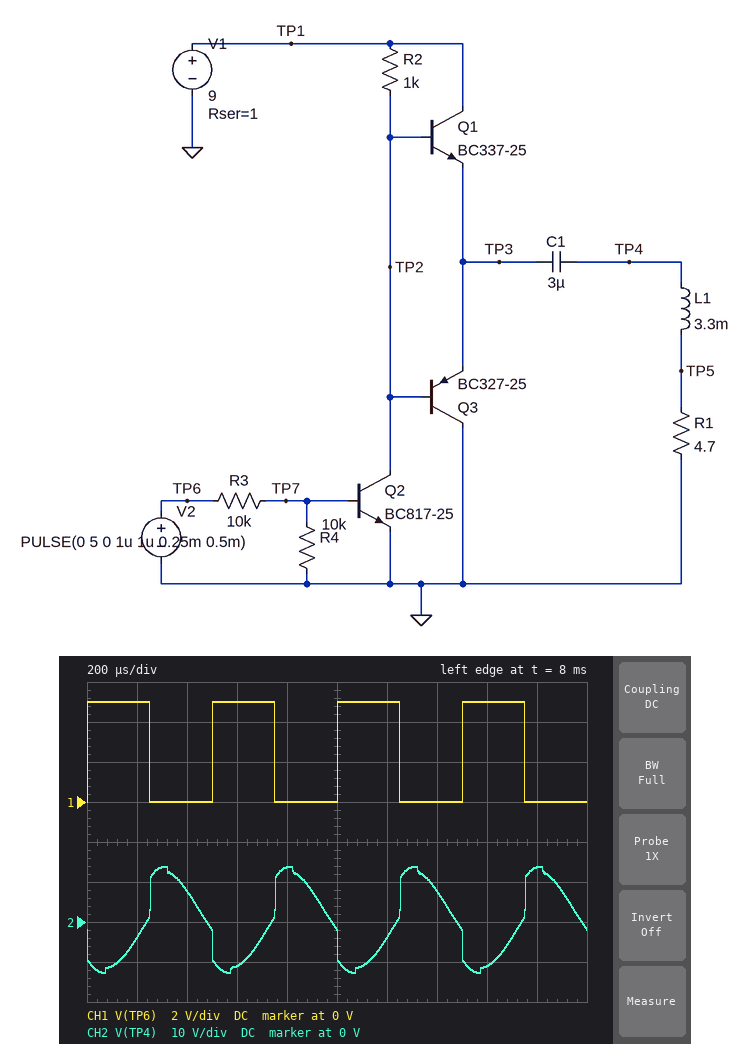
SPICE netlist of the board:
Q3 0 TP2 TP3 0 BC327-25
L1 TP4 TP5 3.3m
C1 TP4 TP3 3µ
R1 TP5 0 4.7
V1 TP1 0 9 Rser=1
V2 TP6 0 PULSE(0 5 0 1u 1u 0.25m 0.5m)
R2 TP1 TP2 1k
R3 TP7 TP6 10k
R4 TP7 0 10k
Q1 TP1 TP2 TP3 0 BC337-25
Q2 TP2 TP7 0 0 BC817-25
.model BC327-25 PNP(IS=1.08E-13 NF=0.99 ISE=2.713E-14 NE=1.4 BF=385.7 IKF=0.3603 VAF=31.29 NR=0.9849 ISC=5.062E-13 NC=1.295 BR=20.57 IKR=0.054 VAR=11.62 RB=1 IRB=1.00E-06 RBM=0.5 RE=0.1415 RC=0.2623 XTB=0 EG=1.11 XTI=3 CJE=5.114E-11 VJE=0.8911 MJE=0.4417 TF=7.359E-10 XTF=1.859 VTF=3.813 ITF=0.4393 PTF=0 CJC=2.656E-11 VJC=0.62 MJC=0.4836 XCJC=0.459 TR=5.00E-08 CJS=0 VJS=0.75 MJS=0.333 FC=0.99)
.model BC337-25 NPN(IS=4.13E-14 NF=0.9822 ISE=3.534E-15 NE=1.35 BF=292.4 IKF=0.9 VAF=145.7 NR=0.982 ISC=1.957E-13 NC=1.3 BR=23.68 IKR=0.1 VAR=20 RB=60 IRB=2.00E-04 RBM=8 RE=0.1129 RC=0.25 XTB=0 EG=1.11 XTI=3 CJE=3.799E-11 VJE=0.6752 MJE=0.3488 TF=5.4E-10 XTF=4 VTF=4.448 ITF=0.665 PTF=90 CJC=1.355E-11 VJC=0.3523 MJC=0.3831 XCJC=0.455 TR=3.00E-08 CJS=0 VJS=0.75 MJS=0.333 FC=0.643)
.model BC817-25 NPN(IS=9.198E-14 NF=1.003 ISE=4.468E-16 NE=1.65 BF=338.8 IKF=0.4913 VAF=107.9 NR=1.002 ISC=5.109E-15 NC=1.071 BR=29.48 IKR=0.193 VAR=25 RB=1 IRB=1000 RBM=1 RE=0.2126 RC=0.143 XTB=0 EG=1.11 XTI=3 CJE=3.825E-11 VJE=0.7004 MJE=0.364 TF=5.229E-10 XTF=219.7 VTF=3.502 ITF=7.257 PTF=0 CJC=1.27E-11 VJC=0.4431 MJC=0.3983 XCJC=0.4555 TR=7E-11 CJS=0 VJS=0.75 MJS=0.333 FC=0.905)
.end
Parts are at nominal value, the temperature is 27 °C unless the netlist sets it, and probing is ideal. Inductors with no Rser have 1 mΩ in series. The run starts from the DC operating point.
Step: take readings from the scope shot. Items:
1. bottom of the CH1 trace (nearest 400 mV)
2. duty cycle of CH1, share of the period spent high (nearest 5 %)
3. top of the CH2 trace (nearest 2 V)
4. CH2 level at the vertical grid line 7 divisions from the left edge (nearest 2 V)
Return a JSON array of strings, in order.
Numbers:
["0 V", "50 %", "14 V", "8 V"]
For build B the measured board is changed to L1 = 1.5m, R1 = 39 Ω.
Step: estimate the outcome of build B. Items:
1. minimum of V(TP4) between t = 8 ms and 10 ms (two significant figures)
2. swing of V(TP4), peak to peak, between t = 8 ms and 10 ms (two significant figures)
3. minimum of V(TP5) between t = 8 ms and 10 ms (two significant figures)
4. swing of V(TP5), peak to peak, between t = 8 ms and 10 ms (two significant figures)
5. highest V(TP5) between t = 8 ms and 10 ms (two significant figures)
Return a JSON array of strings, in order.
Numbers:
["-8.1 V", "17 V", "-4.7 V", "9.3 V", "4.6 V"]
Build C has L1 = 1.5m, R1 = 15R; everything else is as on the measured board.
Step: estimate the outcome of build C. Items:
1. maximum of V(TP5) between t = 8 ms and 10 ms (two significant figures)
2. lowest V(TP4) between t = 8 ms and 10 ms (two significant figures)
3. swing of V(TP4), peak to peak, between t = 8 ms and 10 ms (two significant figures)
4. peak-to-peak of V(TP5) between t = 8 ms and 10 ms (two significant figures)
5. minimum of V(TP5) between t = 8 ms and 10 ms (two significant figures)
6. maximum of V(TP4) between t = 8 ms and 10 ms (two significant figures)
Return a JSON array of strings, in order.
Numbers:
["4.0 V", "-9.6 V", "20 V", "8.1 V", "-4.1 V", "10 V"]
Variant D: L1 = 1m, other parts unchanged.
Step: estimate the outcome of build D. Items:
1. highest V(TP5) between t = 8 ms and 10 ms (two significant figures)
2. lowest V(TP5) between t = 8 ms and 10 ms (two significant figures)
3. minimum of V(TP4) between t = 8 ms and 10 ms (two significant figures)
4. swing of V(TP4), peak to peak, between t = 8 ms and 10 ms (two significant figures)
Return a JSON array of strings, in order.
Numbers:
["1.8 V", "-2.0 V", "-9.2 V", "17 V"]
